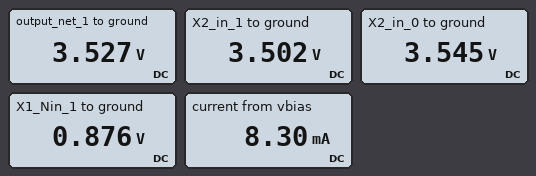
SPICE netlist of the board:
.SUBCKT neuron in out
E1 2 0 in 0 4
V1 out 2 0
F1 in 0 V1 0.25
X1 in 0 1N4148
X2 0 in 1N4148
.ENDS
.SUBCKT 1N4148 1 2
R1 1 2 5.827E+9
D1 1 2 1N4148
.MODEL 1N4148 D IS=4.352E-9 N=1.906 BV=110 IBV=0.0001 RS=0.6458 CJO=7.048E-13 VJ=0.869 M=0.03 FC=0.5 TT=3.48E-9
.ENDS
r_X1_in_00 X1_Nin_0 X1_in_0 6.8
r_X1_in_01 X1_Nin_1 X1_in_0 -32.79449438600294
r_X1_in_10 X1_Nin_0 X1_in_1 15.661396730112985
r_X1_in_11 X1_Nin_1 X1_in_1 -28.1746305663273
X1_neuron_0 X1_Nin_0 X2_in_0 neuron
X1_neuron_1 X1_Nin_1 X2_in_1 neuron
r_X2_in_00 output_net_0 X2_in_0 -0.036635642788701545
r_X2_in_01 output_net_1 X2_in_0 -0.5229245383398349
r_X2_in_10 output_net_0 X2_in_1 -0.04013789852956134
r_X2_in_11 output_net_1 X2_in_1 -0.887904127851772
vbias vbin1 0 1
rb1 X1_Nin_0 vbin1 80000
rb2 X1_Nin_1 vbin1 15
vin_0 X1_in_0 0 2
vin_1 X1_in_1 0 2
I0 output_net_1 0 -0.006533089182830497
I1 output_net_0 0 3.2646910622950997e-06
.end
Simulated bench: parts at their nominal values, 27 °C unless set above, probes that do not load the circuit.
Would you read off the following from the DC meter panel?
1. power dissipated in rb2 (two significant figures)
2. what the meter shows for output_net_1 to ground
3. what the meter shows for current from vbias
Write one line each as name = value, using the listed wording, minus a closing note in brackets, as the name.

power dissipated in rb2 = 1.0 mW
what the meter shows for output_net_1 to ground = 3.527 V
what the meter shows for current from vbias = 8.30 mA
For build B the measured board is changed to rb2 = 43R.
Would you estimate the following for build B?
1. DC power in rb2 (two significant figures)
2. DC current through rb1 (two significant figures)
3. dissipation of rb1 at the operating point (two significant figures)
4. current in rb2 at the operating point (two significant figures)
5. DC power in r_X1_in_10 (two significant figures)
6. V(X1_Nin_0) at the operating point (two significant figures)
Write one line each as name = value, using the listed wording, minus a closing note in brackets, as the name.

DC power in rb2 = 380 µW
DC current through rb1 = 1.5 µA
dissipation of rb1 at the operating point = 170 nW
current in rb2 at the operating point = 3.0 mA
DC power in r_X1_in_10 = 80 mW
V(X1_Nin_0) at the operating point = 880 mV
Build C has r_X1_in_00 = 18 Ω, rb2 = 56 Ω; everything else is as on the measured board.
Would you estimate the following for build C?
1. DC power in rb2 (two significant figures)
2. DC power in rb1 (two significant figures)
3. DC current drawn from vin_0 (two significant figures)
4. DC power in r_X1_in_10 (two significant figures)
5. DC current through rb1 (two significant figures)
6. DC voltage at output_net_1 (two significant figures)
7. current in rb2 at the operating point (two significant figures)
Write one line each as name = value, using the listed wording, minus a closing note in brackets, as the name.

DC power in rb2 = 730 µW
DC power in rb1 = 470 nW
DC current drawn from vin_0 = 30 mA
DC power in r_X1_in_10 = 91 mW
DC current through rb1 = 2.4 µA
DC voltage at output_net_1 = 3.2 V
current in rb2 at the operating point = 3.6 mA
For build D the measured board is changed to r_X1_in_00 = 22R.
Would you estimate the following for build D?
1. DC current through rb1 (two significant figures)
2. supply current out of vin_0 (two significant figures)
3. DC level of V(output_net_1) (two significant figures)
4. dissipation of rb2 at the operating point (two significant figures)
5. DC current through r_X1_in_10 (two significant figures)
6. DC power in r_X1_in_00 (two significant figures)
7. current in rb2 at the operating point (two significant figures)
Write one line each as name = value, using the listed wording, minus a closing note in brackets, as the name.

DC current through rb1 = 2.5 µA
supply current out of vin_0 = 18 mA
DC level of V(output_net_1) = 3.2 V
dissipation of rb2 at the operating point = 2.8 mW
DC current through r_X1_in_10 = 76 mA
DC power in r_X1_in_00 = 65 mW
current in rb2 at the operating point = 14 mA
